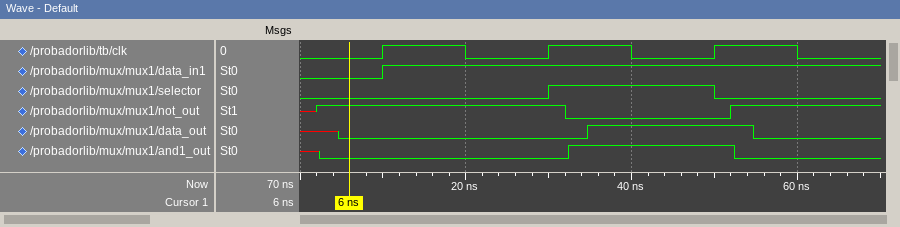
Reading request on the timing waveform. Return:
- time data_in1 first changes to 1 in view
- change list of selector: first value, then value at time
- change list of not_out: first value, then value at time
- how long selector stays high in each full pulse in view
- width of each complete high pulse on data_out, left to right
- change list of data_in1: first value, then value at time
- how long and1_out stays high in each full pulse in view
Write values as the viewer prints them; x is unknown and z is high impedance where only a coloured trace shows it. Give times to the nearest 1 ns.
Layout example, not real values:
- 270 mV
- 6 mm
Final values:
- 10 ns
- 0, 1 at 30 ns, 0 at 50 ns
- x, 1 at 2 ns, 0 at 32 ns, 1 at 52 ns
- 20 ns
- 20 ns
- 0, 1 at 10 ns
- 20 ns
